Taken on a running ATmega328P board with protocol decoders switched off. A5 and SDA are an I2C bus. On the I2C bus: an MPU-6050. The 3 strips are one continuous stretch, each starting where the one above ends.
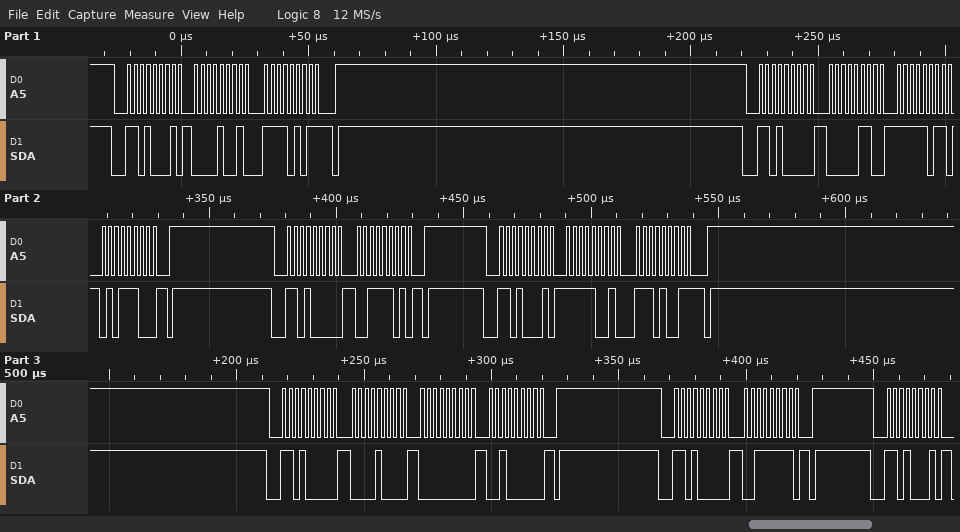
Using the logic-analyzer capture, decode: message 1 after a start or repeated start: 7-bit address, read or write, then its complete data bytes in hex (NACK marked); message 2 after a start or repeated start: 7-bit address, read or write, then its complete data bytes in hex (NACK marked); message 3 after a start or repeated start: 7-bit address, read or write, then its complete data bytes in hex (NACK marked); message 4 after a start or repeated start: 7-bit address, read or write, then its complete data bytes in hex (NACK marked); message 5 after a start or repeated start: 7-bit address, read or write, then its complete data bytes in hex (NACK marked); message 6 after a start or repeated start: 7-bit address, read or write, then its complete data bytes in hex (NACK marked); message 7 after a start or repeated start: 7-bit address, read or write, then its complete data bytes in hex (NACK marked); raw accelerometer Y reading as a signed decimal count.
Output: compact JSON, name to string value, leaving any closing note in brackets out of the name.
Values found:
{"message 1 after a start or repeated start: 7-bit address, read or write, then its complete data bytes in hex": "0x68 read: 09 F5 NACK", "message 2 after a start or repeated start: 7-bit address, read or write, then its complete data bytes in hex": "0x68 write: 06 FB 5C", "message 3 after a start or repeated start: 7-bit address, read or write, then its complete data bytes in hex": "0x68 write: 3D", "message 4 after a start or repeated start: 7-bit address, read or write, then its complete data bytes in hex": "0x68 read: F9 E9 NACK", "message 5 after a start or repeated start: 7-bit address, read or write, then its complete data bytes in hex": "0x68 write: 08 00 20", "message 6 after a start or repeated start: 7-bit address, read or write, then its complete data bytes in hex": "0x68 write: 3F", "message 7 after a start or repeated start: 7-bit address, read or write, then its complete data bytes in hex": "0x68 read", "raw accelerometer Y reading as a signed decimal count": "-1559"}
